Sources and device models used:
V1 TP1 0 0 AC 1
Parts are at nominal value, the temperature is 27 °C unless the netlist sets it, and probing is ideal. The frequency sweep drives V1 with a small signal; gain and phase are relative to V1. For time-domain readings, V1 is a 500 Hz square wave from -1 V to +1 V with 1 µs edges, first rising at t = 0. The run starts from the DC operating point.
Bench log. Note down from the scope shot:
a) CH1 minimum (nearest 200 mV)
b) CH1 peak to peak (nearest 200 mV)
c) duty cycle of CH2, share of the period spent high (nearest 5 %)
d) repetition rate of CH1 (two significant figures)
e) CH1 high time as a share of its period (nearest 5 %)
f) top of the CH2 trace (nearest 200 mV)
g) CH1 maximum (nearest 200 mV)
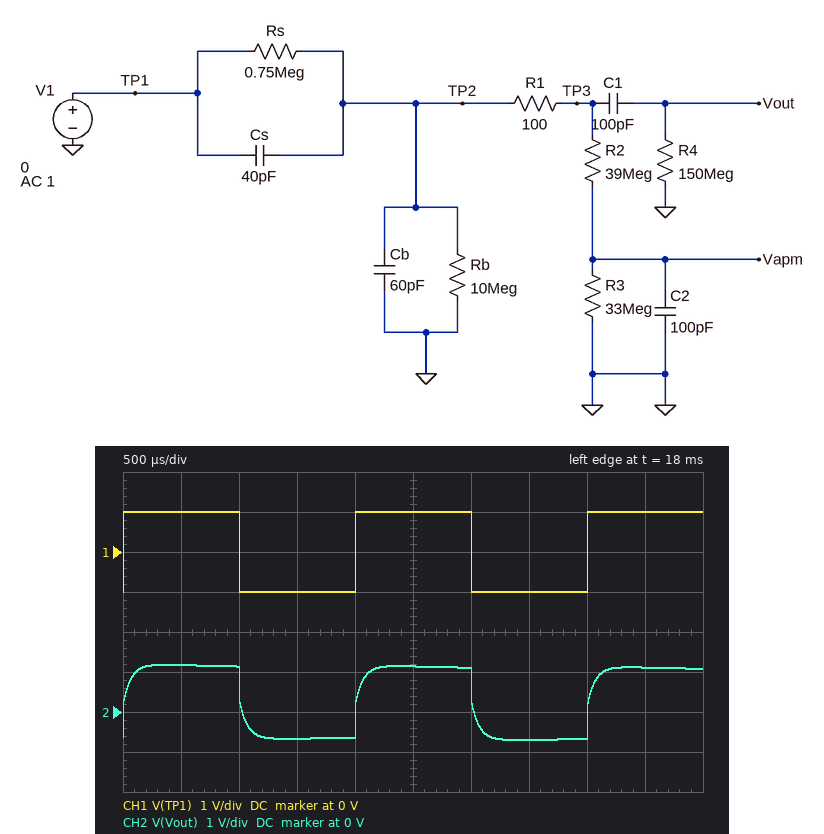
-1.0 V
2.0 V
50 %
500 Hz
50 %
1.2 V
1.0 V
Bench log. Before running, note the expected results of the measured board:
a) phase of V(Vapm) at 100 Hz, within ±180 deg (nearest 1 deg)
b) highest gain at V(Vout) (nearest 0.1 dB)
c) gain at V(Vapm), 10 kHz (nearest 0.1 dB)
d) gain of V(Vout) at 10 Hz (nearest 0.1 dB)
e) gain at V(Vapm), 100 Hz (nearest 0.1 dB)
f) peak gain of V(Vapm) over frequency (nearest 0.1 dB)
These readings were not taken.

-50 deg
-0.8 dB
-54.9 dB
-4.0 dB
-11.1 dB
-7.5 dB
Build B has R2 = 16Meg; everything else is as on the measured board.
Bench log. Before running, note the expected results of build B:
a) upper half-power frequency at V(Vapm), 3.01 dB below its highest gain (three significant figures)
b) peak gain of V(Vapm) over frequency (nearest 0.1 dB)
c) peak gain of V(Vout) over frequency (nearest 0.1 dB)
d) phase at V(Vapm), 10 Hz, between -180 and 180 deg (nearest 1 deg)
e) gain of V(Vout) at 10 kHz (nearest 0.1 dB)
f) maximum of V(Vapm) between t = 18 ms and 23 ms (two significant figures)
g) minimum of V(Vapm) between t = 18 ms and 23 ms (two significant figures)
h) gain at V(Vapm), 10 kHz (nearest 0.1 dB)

142 Hz
-4.2 dB
-0.9 dB
-4 deg
-7.1 dB
250 mV
-250 mV
-47.2 dB
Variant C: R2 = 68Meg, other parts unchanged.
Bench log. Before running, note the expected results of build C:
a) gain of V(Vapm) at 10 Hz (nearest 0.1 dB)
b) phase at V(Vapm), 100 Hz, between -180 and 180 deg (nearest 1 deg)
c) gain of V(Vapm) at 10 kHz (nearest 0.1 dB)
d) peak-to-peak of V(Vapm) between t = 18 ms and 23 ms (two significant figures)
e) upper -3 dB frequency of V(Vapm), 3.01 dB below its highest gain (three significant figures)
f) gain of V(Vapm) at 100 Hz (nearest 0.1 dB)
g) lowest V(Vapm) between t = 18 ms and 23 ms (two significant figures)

-10.5 dB
-56 deg
-59.7 dB
120 mV
70.7 Hz
-15.2 dB
-63 mV
